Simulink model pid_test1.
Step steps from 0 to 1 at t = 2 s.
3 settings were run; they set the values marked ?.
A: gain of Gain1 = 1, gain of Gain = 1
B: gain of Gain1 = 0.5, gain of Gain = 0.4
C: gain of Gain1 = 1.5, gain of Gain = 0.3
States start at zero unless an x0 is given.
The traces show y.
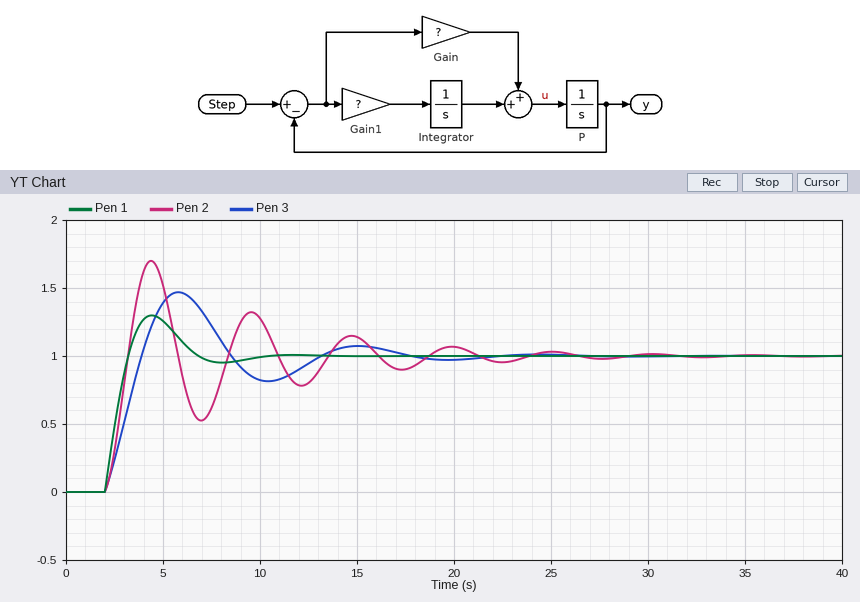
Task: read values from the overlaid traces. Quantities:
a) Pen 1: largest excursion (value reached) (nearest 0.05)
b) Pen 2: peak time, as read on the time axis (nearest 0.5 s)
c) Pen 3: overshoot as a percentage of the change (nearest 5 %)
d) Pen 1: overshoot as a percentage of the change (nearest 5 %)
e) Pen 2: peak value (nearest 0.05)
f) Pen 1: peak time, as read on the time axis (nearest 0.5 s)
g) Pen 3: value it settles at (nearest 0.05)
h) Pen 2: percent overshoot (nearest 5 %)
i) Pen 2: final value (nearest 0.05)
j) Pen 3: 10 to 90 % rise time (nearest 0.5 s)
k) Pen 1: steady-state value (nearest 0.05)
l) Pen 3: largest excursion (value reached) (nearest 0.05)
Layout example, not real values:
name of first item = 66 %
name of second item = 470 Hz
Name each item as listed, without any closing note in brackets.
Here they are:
Pen 1: largest excursion (value reached) = 1.30
Pen 2: peak time, as read on the time axis = 4.5 s
Pen 3: overshoot as a percentage of the change = 45 %
Pen 1: overshoot as a percentage of the change = 30 %
Pen 2: peak value = 1.70
Pen 1: peak time, as read on the time axis = 4.5 s
Pen 3: value it settles at = 1.00
Pen 2: percent overshoot = 70 %
Pen 2: final value = 1.00
Pen 3: 10 to 90 % rise time = 1.5 s
Pen 1: steady-state value = 1.00
Pen 3: largest excursion (value reached) = 1.45
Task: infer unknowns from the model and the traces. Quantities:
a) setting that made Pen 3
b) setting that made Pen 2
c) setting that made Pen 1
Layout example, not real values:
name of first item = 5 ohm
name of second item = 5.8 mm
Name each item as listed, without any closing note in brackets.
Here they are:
setting that made Pen 3 = B
setting that made Pen 2 = C
setting that made Pen 1 = A
